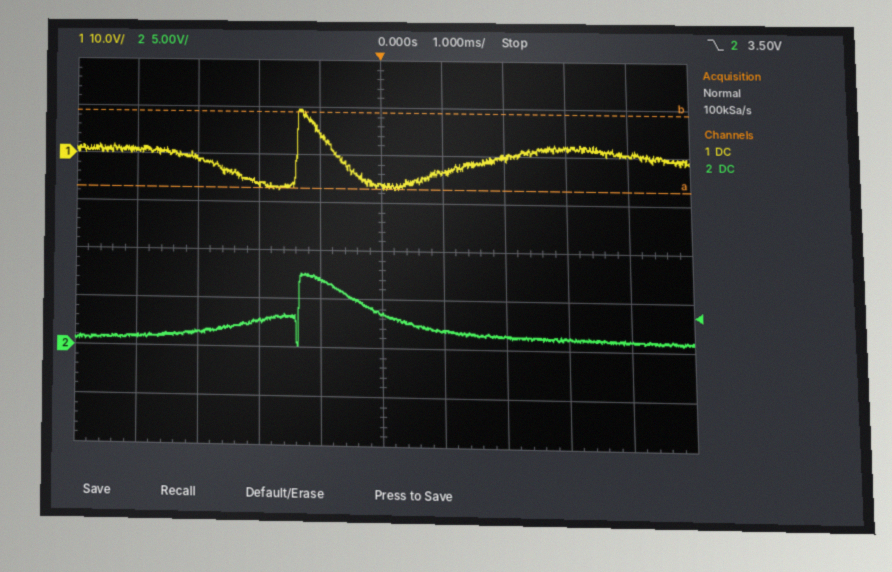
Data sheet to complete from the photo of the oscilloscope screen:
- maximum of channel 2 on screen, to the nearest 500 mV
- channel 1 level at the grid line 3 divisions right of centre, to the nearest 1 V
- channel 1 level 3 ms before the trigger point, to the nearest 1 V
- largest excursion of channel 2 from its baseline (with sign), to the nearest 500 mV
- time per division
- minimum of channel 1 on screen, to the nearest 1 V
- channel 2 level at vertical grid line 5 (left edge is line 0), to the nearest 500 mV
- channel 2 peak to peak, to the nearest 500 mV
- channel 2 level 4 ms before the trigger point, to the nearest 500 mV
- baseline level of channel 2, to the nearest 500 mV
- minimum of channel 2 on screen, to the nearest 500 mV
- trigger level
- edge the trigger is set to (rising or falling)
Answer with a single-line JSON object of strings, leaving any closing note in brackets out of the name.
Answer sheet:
{"maximum of channel 2 on screen, to the nearest 500 mV": "7.5 V", "channel 1 level at the grid line 3 divisions right of centre, to the nearest 1 V": "2 V", "channel 1 level 3 ms before the trigger point, to the nearest 1 V": "-1 V", "largest excursion of channel 2 from its baseline (with sign), to the nearest 500 mV": "+6.5 V", "time per division": "1 ms", "minimum of channel 1 on screen, to the nearest 1 V": "-7 V", "channel 2 level at vertical grid line 5 (left edge is line 0), to the nearest 500 mV": "3.5 V", "channel 2 peak to peak, to the nearest 500 mV": "7.5 V", "channel 2 level 4 ms before the trigger point, to the nearest 500 mV": "1.0 V", "baseline level of channel 2, to the nearest 500 mV": "1.0 V", "minimum of channel 2 on screen, to the nearest 500 mV": "0.0 V", "trigger level": "3.50 V", "edge the trigger is set to": "falling"}
